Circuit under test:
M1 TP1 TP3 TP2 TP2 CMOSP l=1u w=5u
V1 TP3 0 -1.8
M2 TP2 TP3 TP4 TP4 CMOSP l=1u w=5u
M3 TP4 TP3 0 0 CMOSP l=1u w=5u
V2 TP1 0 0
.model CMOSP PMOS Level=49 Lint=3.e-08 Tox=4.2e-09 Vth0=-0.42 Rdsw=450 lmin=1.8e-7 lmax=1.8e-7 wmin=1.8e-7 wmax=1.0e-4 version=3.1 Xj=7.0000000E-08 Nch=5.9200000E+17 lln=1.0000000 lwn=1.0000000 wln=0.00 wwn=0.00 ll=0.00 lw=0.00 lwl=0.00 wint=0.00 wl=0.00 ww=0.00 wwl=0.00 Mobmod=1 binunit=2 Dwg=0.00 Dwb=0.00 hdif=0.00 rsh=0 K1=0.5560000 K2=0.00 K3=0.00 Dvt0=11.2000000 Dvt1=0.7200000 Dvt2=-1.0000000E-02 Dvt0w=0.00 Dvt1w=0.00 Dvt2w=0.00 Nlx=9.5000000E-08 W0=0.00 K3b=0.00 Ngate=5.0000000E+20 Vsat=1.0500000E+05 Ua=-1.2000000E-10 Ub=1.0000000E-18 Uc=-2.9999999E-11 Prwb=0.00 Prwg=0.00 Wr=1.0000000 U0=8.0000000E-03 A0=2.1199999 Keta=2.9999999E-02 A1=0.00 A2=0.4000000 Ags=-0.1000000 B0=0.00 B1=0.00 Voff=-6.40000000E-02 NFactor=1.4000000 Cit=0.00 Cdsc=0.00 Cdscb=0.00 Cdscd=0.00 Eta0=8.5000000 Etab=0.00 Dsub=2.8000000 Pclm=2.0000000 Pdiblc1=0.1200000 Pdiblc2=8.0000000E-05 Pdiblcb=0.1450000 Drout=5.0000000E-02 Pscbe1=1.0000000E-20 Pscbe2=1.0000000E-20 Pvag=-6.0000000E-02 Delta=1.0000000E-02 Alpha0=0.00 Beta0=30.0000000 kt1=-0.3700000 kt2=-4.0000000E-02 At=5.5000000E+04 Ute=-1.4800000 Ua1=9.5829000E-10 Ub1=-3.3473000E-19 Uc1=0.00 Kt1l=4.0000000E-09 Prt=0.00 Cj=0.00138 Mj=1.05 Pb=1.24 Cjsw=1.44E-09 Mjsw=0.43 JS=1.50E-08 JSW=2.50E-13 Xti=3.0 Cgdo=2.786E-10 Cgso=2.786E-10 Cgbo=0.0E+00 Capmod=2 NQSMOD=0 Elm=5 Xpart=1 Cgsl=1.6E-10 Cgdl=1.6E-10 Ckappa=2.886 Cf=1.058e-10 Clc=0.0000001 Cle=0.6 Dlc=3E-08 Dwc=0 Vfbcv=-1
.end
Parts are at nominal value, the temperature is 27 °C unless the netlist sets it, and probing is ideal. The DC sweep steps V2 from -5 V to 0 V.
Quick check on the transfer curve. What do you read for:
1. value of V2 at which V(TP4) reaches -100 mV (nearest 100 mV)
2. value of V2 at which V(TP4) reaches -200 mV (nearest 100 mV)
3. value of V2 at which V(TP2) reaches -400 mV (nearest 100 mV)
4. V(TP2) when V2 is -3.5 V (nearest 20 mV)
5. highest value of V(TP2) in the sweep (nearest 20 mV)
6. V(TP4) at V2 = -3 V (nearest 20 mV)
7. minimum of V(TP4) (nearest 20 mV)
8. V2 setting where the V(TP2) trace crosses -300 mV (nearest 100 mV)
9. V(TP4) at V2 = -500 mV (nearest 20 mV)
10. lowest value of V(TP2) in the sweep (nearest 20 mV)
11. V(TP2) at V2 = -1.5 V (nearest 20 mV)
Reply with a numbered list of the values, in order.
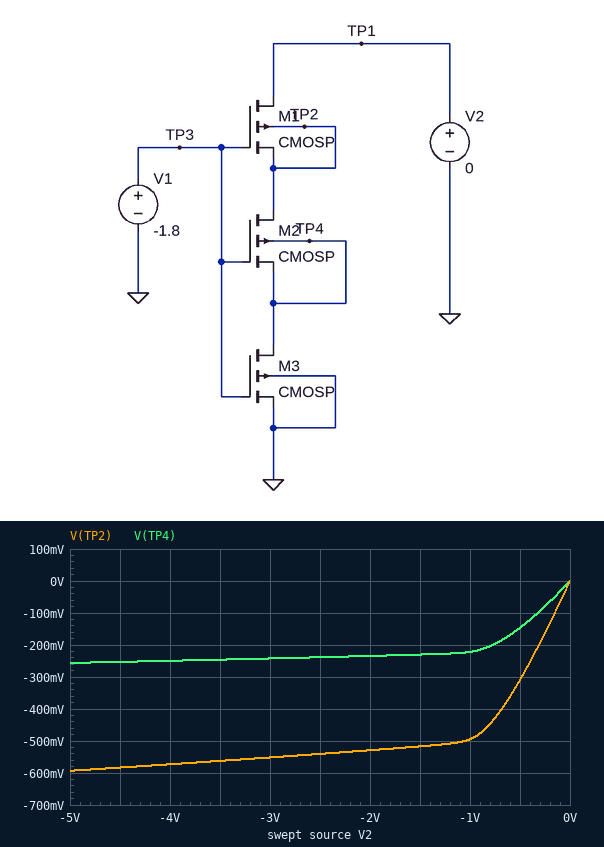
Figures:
1. -300 mV
2. -800 mV
3. -700 mV
4. -560 mV
5. 0 V
6. -240 mV
7. -260 mV
8. -500 mV
9. -140 mV
10. -600 mV
11. -520 mV
